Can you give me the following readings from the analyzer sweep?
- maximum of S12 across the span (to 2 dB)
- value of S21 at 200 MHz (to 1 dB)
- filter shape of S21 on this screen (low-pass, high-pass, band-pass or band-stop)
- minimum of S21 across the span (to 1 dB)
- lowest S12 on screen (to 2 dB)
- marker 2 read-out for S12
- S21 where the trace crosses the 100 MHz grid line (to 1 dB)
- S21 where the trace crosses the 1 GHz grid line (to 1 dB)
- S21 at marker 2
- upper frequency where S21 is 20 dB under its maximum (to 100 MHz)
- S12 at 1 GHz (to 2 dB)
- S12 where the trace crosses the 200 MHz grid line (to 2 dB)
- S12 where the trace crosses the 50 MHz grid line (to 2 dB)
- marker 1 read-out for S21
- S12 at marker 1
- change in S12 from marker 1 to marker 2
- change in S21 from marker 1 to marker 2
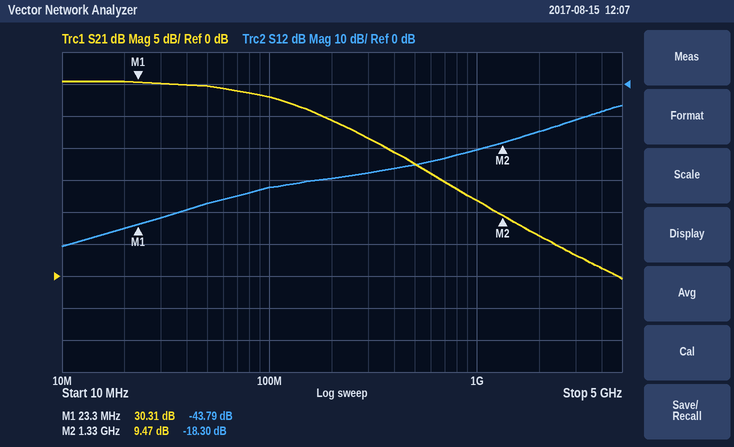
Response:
-6 dB
24 dB
low-pass
0 dB
-50 dB
-18.30 dB
28 dB
12 dB
9.47 dB
1.2 GHz
-20 dB
-30 dB
-38 dB
30.31 dB
-43.79 dB
25.49 dB
-20.84 dB
